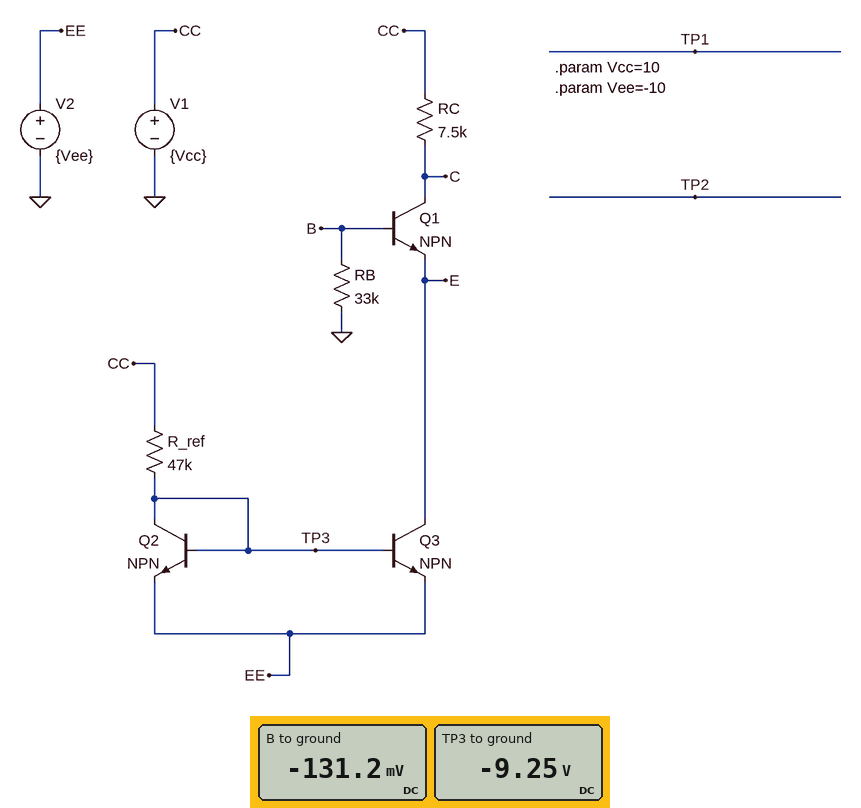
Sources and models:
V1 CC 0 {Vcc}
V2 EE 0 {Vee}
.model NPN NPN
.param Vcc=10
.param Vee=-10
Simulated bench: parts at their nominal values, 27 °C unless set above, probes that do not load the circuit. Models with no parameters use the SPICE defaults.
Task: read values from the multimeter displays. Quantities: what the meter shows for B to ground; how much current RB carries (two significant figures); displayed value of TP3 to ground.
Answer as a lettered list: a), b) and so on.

a) -131.2 mV
b) 4.0 µA
c) -9.25 V
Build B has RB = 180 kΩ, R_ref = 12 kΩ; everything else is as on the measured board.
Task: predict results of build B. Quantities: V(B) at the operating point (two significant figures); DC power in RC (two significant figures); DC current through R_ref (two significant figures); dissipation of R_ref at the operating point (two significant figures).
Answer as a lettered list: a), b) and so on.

a) -2.8 V
b) 18 mW
c) 1.6 mA
d) 31 mW
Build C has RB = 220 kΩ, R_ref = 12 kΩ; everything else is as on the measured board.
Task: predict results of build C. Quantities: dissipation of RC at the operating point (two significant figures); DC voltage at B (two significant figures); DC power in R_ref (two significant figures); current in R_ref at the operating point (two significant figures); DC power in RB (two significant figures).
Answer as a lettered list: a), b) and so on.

a) 18 mW
b) -3.4 V
c) 31 mW
d) 1.6 mA
e) 53 µW
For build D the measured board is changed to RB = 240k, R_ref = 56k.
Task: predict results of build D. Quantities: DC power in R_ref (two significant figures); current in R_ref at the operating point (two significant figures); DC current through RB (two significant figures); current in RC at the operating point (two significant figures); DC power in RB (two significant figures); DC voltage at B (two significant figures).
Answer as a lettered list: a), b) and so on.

a) 6.6 mW
b) 340 µA
c) 3.3 µA
d) 330 µA
e) 2.7 µW
f) -800 mV
